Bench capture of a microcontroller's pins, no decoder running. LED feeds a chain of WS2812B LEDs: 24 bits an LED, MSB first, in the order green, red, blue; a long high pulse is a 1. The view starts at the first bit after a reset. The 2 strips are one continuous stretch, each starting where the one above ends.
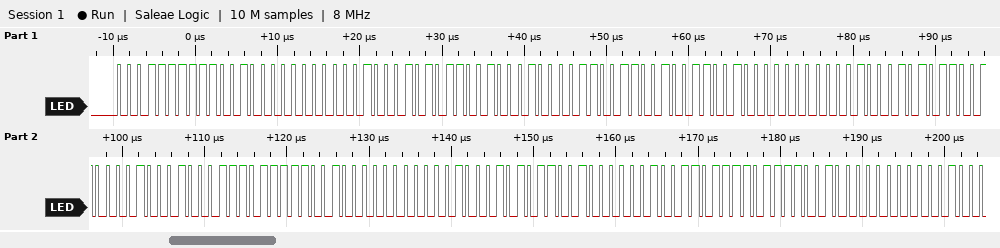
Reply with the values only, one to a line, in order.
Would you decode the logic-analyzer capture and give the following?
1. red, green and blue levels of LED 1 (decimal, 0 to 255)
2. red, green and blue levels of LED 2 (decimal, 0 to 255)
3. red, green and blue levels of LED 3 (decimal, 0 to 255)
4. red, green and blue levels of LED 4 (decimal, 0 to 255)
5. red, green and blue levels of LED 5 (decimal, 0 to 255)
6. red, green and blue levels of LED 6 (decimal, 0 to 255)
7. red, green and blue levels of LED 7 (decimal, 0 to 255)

200, 31, 0
200, 138, 134
200, 100, 0
200, 138, 68
200, 119, 0
200, 138, 19
200, 123, 0
